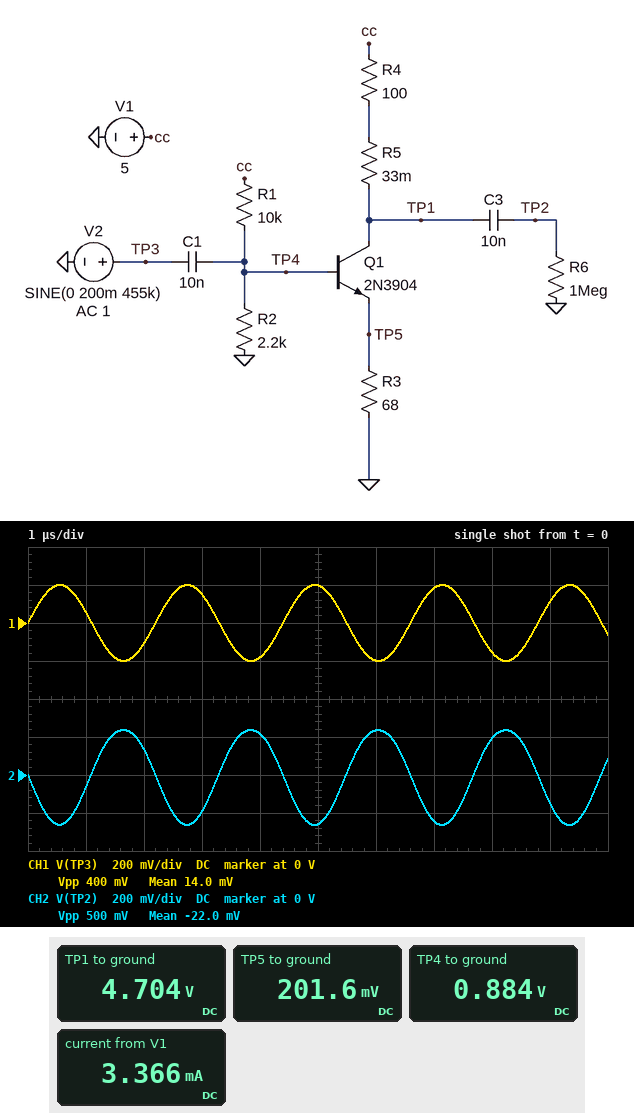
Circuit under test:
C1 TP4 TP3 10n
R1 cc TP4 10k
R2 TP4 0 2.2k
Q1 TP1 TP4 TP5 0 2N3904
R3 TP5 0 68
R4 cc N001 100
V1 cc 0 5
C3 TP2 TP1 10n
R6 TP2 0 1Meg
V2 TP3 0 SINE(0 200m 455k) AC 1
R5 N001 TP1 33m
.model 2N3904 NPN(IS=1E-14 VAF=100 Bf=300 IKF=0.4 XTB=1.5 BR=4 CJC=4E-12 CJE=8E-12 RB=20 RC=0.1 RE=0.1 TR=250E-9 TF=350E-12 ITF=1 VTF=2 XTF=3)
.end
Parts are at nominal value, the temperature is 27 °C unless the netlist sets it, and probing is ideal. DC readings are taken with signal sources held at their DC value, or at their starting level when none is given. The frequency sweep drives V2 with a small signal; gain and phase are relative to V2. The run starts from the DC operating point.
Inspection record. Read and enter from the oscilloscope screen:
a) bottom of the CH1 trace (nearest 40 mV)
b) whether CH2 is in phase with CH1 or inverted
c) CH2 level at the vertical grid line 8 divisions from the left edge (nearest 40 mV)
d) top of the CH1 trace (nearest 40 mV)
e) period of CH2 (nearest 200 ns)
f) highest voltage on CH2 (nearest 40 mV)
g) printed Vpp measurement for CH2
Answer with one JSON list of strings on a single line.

["-200 mV", "inverted", "200 mV", "200 mV", "2.2 µs", "240 mV", "500 mV"]
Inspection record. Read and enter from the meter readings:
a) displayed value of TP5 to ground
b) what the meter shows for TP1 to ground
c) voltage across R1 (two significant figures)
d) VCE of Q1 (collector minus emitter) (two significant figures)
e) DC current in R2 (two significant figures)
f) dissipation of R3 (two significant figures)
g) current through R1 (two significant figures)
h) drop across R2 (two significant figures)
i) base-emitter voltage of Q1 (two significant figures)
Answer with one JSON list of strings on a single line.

["201.6 mV", "4.704 V", "4.1 V", "4.5 V", "400 µA", "600 µW", "410 µA", "880 mV", "680 mV"]
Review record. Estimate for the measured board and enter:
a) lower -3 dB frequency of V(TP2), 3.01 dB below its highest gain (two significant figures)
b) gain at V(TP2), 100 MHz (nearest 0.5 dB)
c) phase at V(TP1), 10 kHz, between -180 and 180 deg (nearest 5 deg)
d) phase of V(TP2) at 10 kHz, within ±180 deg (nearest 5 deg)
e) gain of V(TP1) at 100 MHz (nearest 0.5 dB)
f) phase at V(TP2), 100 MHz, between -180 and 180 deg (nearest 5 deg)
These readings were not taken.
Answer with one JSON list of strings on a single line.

["9.5 kHz", "2.0 dB", "-135 deg", "-135 deg", "2.0 dB", "145 deg"]
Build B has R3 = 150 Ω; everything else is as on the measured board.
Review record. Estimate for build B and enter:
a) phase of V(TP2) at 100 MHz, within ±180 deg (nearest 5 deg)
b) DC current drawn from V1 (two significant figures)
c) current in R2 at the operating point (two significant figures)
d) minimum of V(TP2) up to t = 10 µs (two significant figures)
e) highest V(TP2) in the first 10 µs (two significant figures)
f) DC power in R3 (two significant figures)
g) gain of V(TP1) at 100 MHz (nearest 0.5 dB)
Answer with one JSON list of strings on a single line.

["140 deg", "1.9 mA", "410 µA", "-120 mV", "110 mV", "350 µW", "-4.5 dB"]
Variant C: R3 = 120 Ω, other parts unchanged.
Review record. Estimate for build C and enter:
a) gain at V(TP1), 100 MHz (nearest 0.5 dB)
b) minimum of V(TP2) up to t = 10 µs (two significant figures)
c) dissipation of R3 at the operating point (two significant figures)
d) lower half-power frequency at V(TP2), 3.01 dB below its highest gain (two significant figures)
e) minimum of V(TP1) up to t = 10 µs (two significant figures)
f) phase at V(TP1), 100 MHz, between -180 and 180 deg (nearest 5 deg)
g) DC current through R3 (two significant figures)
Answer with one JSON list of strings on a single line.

["-2.5 dB", "-150 mV", "410 µW", "9.2 kHz", "4.7 V", "140 deg", "1.8 mA"]
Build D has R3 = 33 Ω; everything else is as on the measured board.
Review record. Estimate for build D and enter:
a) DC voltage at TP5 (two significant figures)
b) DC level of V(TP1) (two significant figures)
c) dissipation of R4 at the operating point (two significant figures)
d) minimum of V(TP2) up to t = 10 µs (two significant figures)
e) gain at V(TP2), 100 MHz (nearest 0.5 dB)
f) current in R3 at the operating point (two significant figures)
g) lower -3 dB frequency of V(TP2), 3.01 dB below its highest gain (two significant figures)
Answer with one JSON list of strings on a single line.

["170 mV", "4.5 V", "2.7 mW", "-530 mV", "7.5 dB", "5.2 mA", "10 kHz"]
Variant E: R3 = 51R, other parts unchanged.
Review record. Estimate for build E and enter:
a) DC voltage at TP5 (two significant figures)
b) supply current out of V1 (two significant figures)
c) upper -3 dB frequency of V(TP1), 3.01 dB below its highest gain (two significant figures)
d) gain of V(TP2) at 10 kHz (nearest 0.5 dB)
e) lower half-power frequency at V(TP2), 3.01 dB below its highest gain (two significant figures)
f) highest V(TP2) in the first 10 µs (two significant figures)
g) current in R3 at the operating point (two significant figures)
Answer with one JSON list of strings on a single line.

["190 mV", "4.1 mA", "290 MHz", "2.0 dB", "9.7 kHz", "310 mV", "3.7 mA"]
